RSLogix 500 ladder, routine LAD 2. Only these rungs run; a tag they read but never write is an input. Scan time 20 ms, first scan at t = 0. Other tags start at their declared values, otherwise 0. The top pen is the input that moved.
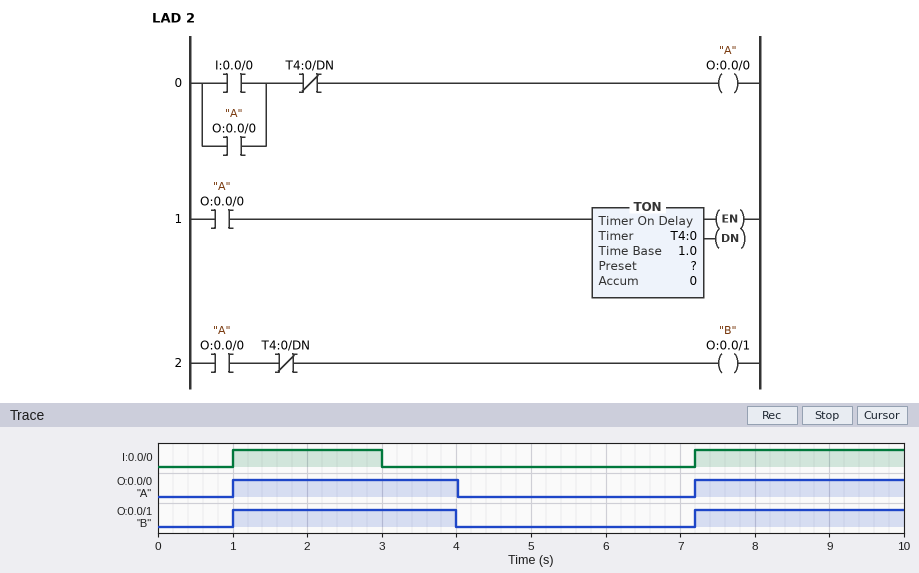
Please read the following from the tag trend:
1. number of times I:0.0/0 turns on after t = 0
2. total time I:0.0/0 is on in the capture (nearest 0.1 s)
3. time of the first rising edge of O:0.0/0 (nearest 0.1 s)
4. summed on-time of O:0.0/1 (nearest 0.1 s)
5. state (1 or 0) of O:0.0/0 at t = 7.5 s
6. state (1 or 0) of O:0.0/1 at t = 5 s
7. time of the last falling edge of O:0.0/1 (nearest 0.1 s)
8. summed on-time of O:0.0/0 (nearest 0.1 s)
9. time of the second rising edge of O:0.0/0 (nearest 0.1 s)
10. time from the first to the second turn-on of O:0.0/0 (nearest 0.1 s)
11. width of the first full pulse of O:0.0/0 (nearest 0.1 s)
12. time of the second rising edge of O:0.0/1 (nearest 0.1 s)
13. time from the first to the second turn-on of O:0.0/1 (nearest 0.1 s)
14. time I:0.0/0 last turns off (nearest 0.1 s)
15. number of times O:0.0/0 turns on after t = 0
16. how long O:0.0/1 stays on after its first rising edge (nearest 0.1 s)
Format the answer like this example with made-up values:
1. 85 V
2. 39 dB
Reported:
1. 2
2. 4.8 s
3. 1.0 s
4. 5.8 s
5. 1
6. 0
7. 4.0 s
8. 5.8 s
9. 7.2 s
10. 6.2 s
11. 3.0 s
12. 7.2 s
13. 6.2 s
14. 3.0 s
15. 2
16. 3.0 s
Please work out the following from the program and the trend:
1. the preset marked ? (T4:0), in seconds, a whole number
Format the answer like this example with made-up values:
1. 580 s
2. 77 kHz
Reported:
1. 3 s
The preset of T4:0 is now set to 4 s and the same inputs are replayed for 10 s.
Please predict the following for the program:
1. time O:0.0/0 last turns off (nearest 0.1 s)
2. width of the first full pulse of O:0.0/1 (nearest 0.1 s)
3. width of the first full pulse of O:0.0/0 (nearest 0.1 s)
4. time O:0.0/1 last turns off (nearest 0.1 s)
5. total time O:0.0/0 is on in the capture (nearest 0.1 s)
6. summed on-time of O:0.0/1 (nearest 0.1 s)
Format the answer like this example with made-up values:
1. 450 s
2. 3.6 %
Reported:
1. 5.0 s
2. 4.0 s
3. 4.0 s
4. 5.0 s
5. 6.8 s
6. 6.8 s
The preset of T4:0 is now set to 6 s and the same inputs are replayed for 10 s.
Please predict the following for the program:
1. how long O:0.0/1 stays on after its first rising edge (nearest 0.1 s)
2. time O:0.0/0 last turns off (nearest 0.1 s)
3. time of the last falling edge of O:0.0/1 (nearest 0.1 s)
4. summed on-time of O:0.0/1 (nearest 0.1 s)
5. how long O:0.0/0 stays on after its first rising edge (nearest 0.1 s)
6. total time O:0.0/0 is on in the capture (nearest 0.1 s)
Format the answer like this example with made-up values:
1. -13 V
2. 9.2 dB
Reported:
1. 6.0 s
2. 7.0 s
3. 7.0 s
4. 8.8 s
5. 6.0 s
6. 8.8 s
